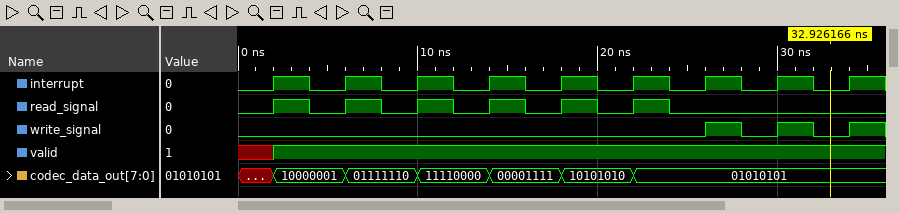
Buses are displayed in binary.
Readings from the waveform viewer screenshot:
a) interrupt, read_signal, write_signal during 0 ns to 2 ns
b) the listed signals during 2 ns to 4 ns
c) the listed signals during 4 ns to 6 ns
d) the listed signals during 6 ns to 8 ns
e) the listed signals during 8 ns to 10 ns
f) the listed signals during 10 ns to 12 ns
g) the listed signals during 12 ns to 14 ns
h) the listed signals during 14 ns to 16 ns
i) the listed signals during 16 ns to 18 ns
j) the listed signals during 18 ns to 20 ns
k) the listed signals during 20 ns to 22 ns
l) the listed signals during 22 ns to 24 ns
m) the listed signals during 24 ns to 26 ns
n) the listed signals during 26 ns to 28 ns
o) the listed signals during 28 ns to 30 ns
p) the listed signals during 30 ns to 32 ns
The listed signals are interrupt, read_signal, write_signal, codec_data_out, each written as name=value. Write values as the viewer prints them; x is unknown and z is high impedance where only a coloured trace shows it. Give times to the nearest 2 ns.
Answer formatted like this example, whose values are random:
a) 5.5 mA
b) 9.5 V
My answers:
a) interrupt=0, read_signal=0, write_signal=0
b) interrupt=1, read_signal=1, write_signal=0, codec_data_out=10000001
c) interrupt=0, read_signal=0, write_signal=0, codec_data_out=10000001
d) interrupt=1, read_signal=1, write_signal=0, codec_data_out=01111110
e) interrupt=0, read_signal=0, write_signal=0, codec_data_out=01111110
f) interrupt=1, read_signal=1, write_signal=0, codec_data_out=11110000
g) interrupt=0, read_signal=0, write_signal=0, codec_data_out=11110000
h) interrupt=1, read_signal=1, write_signal=0, codec_data_out=00001111
i) interrupt=0, read_signal=0, write_signal=0, codec_data_out=00001111
j) interrupt=1, read_signal=1, write_signal=0, codec_data_out=10101010
k) interrupt=0, read_signal=0, write_signal=0, codec_data_out=10101010
l) interrupt=1, read_signal=1, write_signal=0, codec_data_out=01010101
m) interrupt=0, read_signal=0, write_signal=0, codec_data_out=01010101
n) interrupt=1, read_signal=0, write_signal=1, codec_data_out=01010101
o) interrupt=0, read_signal=0, write_signal=0, codec_data_out=01010101
p) interrupt=1, read_signal=0, write_signal=1, codec_data_out=01010101
